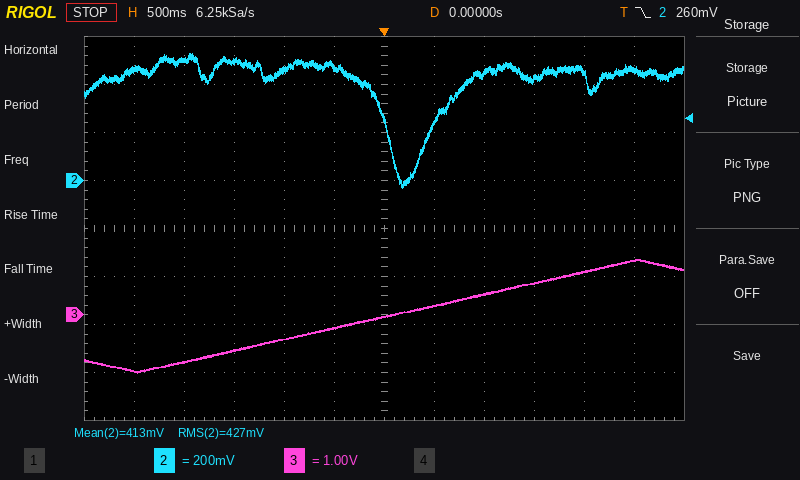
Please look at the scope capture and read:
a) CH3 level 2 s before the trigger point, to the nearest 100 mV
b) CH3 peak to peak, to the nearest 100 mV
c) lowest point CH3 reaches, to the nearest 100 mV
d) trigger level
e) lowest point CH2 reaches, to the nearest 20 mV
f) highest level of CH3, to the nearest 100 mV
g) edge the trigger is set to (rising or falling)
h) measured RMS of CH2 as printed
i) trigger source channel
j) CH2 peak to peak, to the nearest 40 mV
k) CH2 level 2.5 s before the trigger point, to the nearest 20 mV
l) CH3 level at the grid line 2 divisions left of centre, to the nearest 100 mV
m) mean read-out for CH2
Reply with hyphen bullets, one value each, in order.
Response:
- -1.0 V
- 2.4 V
- -1.2 V
- 260 mV
- -40 mV
- 1.2 V
- falling
- 427 mV
- CH2
- 560 mV
- 460 mV
- -500 mV
- 413 mV
